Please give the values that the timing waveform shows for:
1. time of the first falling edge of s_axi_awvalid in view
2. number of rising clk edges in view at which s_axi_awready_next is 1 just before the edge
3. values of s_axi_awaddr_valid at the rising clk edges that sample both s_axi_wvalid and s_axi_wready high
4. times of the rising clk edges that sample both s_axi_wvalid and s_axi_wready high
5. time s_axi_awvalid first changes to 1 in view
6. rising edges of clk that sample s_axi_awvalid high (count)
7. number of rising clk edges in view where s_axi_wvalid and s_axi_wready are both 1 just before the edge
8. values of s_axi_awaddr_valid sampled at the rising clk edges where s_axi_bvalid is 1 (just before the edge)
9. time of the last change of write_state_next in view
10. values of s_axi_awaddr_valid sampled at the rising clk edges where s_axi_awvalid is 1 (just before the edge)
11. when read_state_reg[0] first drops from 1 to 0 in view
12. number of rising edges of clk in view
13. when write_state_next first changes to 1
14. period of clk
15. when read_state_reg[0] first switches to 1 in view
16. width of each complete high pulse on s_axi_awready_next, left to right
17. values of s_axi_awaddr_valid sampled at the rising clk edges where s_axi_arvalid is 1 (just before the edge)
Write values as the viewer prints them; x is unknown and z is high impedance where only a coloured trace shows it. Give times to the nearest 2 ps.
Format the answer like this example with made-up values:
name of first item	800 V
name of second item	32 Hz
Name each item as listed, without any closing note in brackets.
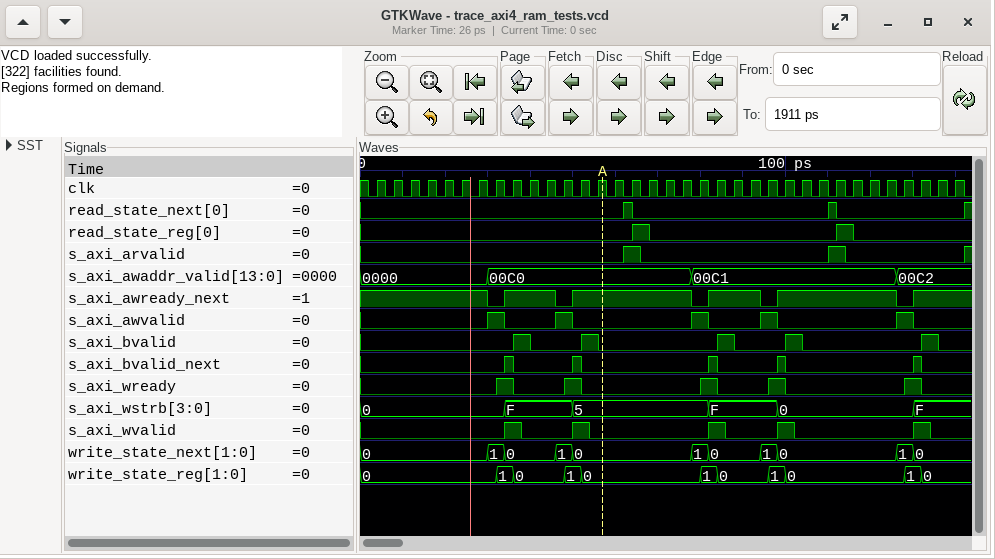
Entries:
time of the first falling edge of s_axi_awvalid in view	34 ps
number of rising clk edges in view at which s_axi_awready_next is 1 just before the edge	30
values of s_axi_awaddr_valid at the rising clk edges that sample both s_axi_wvalid and s_axi_wready high	00C0, 00C0, 00C1, 00C1, 00C2
times of the rising clk edges that sample both s_axi_wvalid and s_axi_wready high	36 ps, 52 ps, 84 ps, 100 ps, 132 ps
time s_axi_awvalid first changes to 1 in view	30 ps
rising edges of clk that sample s_axi_awvalid high	5
number of rising clk edges in view where s_axi_wvalid and s_axi_wready are both 1 just before the edge	5
values of s_axi_awaddr_valid sampled at the rising clk edges where s_axi_bvalid is 1	00C0, 00C0, 00C1, 00C1, 00C2
time of the last change of write_state_next in view	130 ps
values of s_axi_awaddr_valid sampled at the rising clk edges where s_axi_awvalid is 1	00C0, 00C0, 00C1, 00C1, 00C2
when read_state_reg[0] first drops from 1 to 0 in view	68 ps
number of rising edges of clk in view	35
when write_state_next first changes to 1	30 ps
period of clk	4 ps
when read_state_reg[0] first switches to 1 in view	64 ps
width of each complete high pulse on s_axi_awready_next, left to right	12 ps, 28 ps, 12 ps, 28 ps
values of s_axi_awaddr_valid sampled at the rising clk edges where s_axi_arvalid is 1	00C0, 00C1
